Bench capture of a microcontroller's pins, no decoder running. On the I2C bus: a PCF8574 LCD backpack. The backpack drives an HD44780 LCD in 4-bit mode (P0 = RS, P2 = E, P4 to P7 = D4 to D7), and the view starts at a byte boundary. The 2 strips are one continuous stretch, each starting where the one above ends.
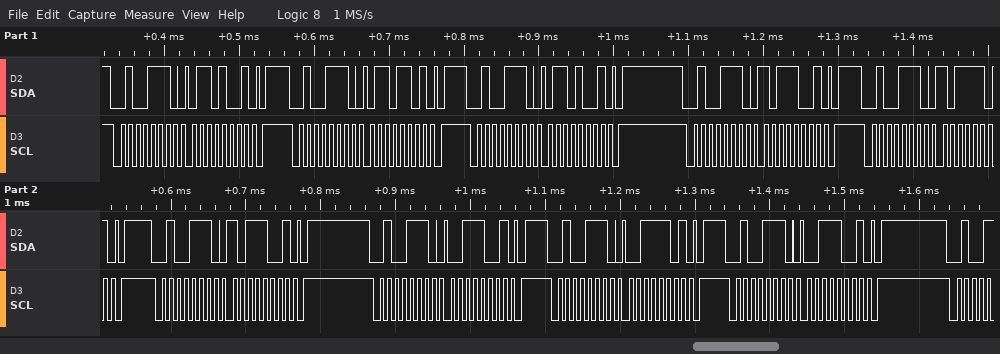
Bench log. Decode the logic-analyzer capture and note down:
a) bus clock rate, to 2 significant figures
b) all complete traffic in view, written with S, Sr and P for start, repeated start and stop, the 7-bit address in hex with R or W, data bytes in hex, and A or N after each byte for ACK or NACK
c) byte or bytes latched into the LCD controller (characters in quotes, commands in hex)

100 kHz
S 27W A 69 A P S 27W A 6D A P S 27W A 69 A P S 27W A B9 A P S 27W A BD A P S 27W A B9 A P S 27W A 39 A P S 27W A 3D A P S 27W A 39 A P
'k'
